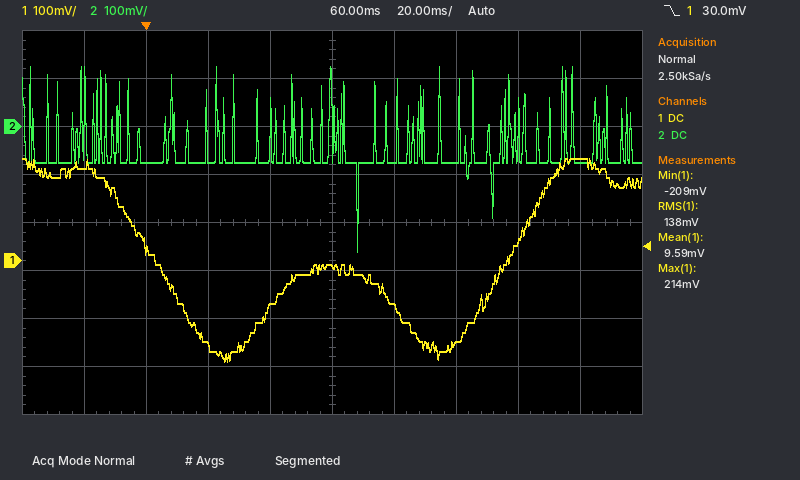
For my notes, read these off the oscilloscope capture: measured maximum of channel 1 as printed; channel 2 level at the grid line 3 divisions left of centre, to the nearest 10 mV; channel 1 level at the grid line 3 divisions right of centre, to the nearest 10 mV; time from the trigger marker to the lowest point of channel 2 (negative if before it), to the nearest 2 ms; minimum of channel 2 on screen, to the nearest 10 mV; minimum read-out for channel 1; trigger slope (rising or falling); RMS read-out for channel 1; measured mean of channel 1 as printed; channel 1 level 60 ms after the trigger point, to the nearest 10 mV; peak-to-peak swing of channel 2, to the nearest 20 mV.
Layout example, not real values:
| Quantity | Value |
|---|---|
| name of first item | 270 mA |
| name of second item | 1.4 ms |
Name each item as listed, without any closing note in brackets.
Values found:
| Quantity | Value |
|---|---|
| measured maximum of channel 1 as printed | 214 mV |
| channel 2 level at the grid line 3 divisions left of centre, to the nearest 10 mV | -80 mV |
| channel 1 level at the grid line 3 divisions right of centre, to the nearest 10 mV | 40 mV |
| time from the trigger marker to the lowest point of channel 2 (negative if before it), to the nearest 2 ms | +68 ms |
| minimum of channel 2 on screen, to the nearest 10 mV | -260 mV |
| minimum read-out for channel 1 | -209 mV |
| trigger slope | falling |
| RMS read-out for channel 1 | 138 mV |
| measured mean of channel 1 as printed | 9.59 mV |
| channel 1 level 60 ms after the trigger point, to the nearest 10 mV | -10 mV |
| peak-to-peak swing of channel 2, to the nearest 20 mV | 380 mV |
